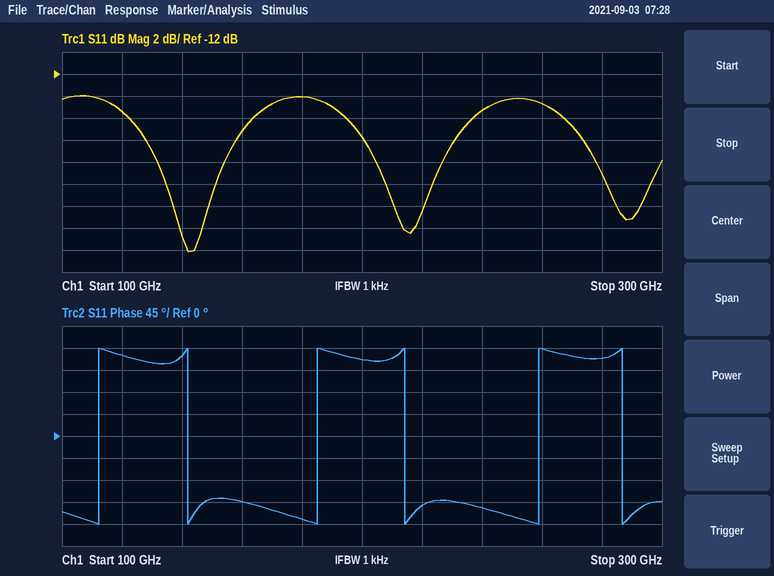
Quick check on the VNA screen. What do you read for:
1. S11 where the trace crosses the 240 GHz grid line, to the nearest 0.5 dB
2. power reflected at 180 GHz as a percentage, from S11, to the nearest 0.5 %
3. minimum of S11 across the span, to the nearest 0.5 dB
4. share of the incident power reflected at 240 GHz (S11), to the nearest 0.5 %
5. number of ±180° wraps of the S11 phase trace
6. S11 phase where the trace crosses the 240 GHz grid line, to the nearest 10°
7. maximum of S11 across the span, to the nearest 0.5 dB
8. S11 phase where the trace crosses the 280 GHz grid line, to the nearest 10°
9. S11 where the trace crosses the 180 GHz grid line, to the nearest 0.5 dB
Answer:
-15.5 dB
4.0 %
-28.0 dB
3.0 %
6
-150°
-14.0 dB
160°
-14.0 dB
